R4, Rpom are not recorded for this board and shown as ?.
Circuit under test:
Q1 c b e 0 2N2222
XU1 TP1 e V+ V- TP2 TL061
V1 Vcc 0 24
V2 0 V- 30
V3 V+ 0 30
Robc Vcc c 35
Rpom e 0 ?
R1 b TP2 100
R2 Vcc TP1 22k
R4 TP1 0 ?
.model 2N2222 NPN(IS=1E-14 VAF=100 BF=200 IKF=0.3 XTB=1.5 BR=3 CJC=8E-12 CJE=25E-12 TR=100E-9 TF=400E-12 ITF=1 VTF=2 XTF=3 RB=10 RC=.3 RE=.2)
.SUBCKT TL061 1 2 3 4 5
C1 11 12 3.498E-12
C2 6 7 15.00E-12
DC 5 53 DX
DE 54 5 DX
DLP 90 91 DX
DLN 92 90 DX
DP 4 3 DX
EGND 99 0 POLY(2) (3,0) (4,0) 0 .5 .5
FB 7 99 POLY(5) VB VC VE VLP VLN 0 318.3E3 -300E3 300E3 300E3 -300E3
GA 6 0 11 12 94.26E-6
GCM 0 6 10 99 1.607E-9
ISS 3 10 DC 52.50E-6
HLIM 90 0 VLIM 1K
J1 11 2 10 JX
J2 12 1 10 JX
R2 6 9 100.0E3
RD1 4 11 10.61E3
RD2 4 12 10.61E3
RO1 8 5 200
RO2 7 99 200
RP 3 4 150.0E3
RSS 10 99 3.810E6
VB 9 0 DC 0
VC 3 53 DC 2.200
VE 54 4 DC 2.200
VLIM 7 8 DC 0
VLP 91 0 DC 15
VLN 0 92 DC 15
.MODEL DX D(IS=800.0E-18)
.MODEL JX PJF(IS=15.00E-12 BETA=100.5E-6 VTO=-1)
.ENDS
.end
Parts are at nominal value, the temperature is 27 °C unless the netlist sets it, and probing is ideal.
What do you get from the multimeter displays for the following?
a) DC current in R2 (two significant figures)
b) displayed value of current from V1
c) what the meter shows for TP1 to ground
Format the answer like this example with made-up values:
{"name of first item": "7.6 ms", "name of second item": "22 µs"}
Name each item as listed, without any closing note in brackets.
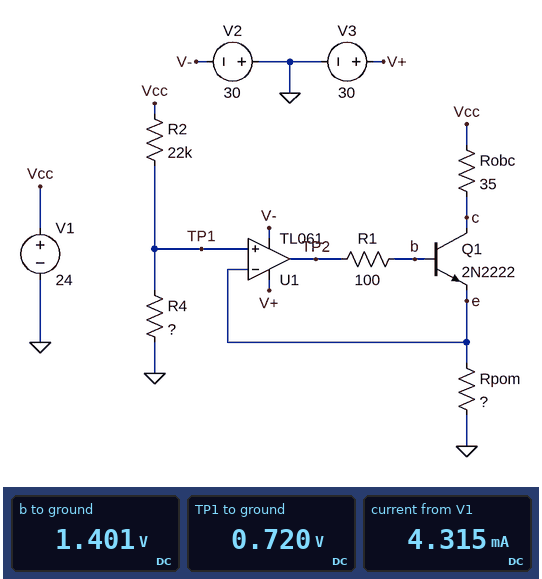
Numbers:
{"DC current in R2": "1.1 mA", "displayed value of current from V1": "4.315 mA", "what the meter shows for TP1 to ground": "0.720 V"}
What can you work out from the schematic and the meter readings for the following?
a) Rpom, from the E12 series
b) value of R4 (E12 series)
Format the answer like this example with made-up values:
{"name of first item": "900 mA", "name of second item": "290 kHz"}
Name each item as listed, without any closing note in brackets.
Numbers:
{"Rpom, from the E12 series": "220 Ω", "value of R4": "680 Ω"}
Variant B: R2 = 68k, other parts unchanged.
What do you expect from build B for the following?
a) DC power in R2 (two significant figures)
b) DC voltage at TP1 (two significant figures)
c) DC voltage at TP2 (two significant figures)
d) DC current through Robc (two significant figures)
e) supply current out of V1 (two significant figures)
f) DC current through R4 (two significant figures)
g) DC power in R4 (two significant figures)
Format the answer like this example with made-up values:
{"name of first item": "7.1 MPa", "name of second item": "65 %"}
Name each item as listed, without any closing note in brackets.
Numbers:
{"DC power in R2": "8.3 mW", "DC voltage at TP1": "240 mV", "DC voltage at TP2": "890 mV", "DC current through Robc": "1.1 mA", "supply current out of V1": "1.4 mA", "DC current through R4": "350 µA", "DC power in R4": "83 µW"}
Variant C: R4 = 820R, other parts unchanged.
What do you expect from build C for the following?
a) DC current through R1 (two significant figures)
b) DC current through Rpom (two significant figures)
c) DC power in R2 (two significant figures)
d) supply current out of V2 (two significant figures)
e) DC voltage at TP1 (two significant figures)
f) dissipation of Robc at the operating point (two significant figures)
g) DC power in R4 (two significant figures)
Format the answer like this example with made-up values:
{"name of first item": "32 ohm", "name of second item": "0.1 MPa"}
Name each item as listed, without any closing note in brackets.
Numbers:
{"DC current through R1": "16 µA", "DC current through Rpom": "3.9 mA", "DC power in R2": "24 mW", "supply current out of V2": "450 µA", "DC voltage at TP1": "860 mV", "dissipation of Robc at the operating point": "530 µW", "DC power in R4": "910 µW"}
